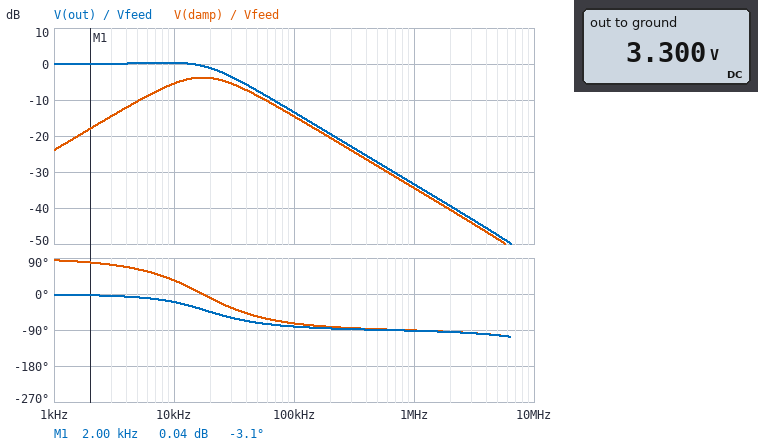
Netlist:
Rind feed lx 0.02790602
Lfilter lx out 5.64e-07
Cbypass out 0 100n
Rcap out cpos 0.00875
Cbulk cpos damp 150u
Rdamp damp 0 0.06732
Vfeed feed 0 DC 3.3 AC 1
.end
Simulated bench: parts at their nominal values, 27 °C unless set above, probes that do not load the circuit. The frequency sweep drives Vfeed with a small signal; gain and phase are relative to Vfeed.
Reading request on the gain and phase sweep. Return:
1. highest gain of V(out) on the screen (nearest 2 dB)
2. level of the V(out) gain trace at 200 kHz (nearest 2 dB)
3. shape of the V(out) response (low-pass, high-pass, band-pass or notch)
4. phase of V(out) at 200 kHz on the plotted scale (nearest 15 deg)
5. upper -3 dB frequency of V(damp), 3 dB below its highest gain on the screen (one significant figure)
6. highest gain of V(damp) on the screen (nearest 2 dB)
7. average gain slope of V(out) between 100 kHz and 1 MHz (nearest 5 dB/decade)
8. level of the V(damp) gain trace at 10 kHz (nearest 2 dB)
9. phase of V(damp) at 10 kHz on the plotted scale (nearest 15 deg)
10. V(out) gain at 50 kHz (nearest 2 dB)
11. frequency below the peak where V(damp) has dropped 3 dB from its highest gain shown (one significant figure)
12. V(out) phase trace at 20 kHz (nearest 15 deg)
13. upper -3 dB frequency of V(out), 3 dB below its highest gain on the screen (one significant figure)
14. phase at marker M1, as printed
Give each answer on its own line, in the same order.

0 dB
-20 dB
low-pass
-90 deg
40 kHz
-4 dB
-20 dB/decade
-6 dB
30 deg
-8 dB
8 kHz
-45 deg
30 kHz
-3.1 deg
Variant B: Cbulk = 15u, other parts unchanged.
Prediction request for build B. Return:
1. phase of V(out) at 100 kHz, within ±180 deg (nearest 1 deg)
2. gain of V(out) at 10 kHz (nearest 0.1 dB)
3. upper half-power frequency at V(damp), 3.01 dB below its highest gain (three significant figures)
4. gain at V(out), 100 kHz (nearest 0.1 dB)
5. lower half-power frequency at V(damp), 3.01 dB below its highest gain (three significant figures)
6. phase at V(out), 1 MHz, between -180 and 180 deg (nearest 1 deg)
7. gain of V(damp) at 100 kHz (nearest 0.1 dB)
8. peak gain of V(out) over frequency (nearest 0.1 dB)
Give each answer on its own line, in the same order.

-122 deg
0.3 dB
71.0 kHz
-6.3 dB
41.9 kHz
-99 deg
-12.1 dB
6.3 dB
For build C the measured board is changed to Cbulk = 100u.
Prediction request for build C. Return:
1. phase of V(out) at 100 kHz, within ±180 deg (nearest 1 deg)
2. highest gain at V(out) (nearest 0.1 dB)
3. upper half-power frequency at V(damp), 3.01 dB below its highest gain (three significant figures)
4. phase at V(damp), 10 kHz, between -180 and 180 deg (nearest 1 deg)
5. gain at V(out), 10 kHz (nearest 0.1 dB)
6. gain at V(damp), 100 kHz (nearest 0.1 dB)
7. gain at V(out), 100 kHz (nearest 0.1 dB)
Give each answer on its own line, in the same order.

-85 deg
1.0 dB
40.4 kHz
50 deg
0.8 dB
-14.4 dB
-13.2 dB
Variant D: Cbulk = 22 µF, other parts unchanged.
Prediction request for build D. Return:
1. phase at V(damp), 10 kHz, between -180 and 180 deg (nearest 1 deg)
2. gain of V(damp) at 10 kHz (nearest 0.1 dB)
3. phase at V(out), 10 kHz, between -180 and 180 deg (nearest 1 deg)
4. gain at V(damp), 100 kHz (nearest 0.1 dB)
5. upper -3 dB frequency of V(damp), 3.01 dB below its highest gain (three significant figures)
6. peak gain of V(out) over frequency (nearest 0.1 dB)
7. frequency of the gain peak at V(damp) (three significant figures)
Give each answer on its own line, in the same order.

81 deg
-20.3 dB
-3 deg
-13.0 dB
62.0 kHz
5.0 dB
45.1 kHz
